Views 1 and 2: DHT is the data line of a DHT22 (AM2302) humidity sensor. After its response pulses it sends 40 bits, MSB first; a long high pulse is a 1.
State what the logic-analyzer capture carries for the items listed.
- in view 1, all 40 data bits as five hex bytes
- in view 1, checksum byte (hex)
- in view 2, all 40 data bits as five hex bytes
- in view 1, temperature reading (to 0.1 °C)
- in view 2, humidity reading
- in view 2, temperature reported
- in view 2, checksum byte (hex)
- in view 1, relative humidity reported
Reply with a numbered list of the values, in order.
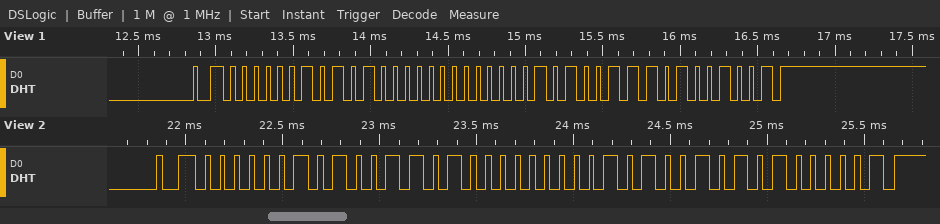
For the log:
1. 02 A0 00 A7 49
2. 0x49
3. 02 9A 00 A5 41
4. 16.7 °C
5. 66.6 %
6. 16.5 °C
7. 0x41
8. 67.2 %
